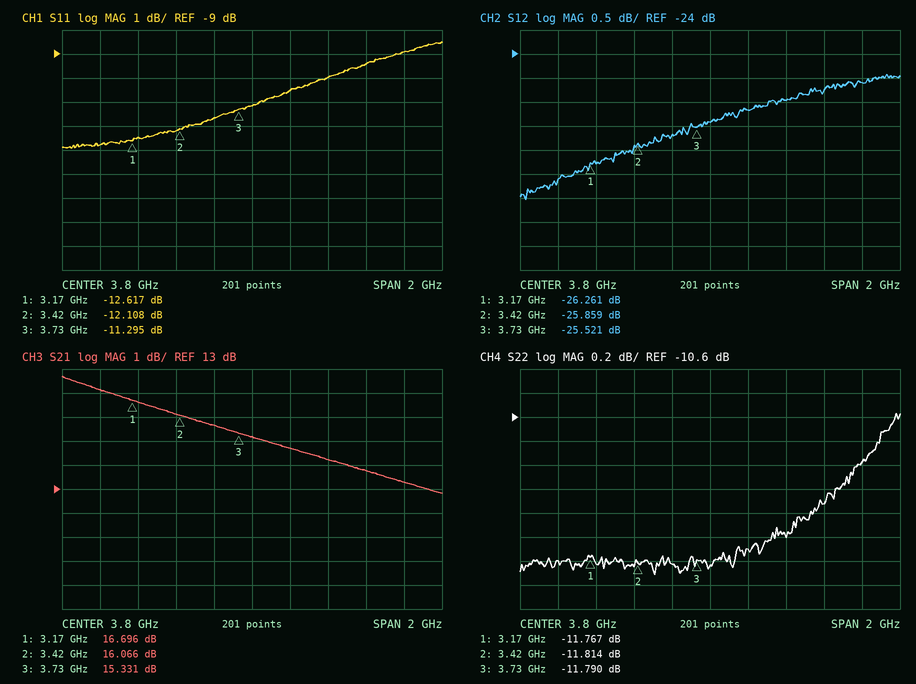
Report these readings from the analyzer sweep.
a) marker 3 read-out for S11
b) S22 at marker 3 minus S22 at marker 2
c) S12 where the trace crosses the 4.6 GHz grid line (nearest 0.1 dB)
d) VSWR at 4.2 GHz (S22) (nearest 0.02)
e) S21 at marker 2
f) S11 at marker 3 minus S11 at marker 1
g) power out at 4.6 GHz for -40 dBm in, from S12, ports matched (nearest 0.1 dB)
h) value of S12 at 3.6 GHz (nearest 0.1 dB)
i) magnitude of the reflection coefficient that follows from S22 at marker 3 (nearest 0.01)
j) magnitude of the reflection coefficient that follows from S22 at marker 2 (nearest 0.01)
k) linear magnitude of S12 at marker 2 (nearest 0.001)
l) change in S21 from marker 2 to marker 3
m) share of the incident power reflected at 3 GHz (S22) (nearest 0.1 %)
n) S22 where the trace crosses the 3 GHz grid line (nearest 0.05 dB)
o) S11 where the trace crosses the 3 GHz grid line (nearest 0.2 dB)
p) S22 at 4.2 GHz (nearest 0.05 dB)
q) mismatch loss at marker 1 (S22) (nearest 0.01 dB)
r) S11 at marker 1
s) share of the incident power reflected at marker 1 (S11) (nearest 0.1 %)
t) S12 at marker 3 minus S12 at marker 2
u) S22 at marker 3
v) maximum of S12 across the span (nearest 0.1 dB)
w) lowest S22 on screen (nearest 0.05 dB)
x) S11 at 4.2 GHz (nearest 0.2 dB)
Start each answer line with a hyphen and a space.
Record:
- -11.295 dB
- 0.024 dB
- -24.6 dB
- 1.72
- 16.066 dB
- 1.322 dB
- -64.6 dBm
- -25.7 dB
- 0.26
- 0.26
- 0.051
- -0.735 dB
- 6.6 %
- -11.80 dB
- -12.8 dB
- -11.60 dB
- 0.30 dB
- -12.617 dB
- 5.5 %
- 0.338 dB
- -11.790 dB
- -24.4 dB
- -11.90 dB
- -10.0 dB
